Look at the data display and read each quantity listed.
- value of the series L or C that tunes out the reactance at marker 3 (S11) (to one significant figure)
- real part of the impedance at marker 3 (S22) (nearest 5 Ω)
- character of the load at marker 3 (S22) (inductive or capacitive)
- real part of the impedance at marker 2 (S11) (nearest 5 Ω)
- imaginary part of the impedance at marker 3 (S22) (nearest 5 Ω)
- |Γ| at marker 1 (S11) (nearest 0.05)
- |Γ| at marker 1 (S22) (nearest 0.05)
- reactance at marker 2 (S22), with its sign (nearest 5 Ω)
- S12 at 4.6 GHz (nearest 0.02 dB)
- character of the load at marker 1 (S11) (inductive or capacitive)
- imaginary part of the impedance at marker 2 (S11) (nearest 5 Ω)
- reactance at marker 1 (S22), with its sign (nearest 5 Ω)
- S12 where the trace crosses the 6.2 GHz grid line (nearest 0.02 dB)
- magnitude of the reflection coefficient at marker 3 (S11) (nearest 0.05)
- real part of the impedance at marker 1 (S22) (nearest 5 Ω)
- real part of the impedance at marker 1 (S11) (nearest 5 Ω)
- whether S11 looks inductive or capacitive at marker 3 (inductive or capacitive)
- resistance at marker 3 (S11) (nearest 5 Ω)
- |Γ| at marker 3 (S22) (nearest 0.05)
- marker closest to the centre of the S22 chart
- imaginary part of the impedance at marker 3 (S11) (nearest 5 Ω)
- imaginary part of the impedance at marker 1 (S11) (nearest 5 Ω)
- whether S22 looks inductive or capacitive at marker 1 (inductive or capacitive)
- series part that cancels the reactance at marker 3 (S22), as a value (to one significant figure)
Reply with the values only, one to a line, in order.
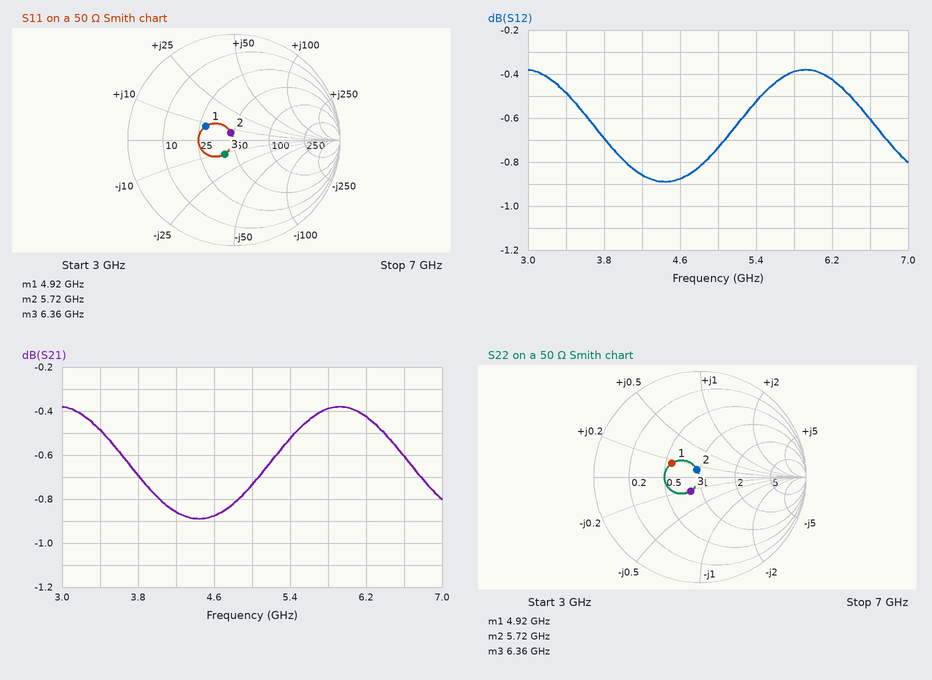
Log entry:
300 pH
40 Ω
capacitive
45 Ω
-10 Ω
0.30
0.30
+5 Ω
-0.88 dB
inductive
+5 Ω
+10 Ω
-0.42 dB
0.15
30 Ω
30 Ω
capacitive
40 Ω
0.15
marker 2
-10 Ω
+10 Ω
inductive
300 pH
